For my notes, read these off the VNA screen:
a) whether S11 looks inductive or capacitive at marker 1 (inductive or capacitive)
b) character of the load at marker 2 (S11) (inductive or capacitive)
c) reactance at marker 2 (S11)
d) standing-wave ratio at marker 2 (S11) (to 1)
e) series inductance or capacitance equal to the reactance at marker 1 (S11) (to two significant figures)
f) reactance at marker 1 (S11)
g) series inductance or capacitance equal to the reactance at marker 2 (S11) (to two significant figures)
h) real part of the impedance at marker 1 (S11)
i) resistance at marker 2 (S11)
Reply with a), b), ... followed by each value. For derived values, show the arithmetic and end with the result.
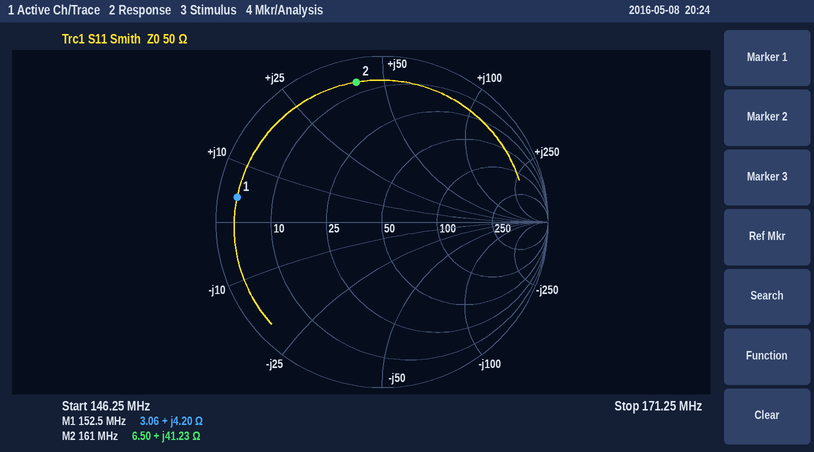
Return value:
a) inductive
b) inductive
c) +41.23 Ω
d) 13
e) L = 4.2 Ω/(2π × 152.5 MHz) ≈ 4.4 nH
f) +4.20 Ω
g) L = 41.23 Ω/(2π × 161 MHz) ≈ 41 nH
h) 3.06 Ω
i) 6.50 Ω
